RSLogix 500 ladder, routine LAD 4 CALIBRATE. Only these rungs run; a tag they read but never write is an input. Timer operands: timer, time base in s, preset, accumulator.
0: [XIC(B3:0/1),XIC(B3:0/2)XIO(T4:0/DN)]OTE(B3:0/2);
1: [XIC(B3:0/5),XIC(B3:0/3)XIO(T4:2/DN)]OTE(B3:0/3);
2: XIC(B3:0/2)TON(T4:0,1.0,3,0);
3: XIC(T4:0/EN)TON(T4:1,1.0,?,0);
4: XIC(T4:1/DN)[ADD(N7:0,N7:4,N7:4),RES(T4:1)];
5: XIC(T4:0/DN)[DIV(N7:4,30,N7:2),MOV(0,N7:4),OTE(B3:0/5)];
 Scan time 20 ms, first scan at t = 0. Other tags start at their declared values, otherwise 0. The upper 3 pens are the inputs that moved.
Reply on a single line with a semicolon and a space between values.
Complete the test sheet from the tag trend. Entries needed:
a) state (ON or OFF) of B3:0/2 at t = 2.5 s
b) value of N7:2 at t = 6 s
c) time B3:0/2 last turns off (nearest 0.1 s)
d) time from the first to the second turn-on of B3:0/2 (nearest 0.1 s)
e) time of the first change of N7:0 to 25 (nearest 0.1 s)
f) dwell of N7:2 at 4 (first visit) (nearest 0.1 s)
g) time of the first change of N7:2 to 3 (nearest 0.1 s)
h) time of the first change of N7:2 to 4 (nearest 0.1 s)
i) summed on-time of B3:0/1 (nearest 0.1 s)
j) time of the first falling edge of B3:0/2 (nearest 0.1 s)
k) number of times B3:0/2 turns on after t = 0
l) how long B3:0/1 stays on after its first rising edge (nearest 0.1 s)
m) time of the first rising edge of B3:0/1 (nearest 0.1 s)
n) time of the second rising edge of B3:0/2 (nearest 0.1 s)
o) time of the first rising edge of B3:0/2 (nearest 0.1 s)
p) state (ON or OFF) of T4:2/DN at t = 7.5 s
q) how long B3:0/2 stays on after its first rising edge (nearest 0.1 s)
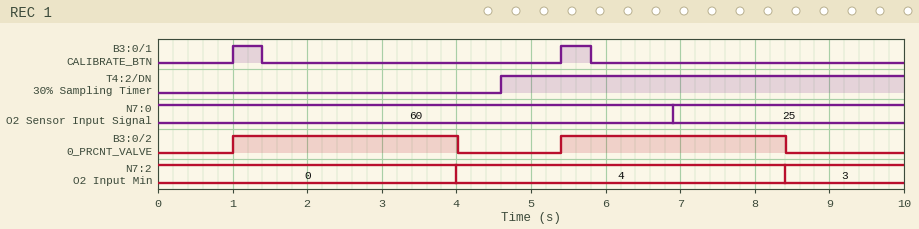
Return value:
ON; 4; 8.4 s; 4.4 s; 6.9 s; 4.4 s; 8.4 s; 4.0 s; 0.8 s; 4.0 s; 2; 0.4 s; 1.0 s; 5.4 s; 1.0 s; ON; 3.0 s
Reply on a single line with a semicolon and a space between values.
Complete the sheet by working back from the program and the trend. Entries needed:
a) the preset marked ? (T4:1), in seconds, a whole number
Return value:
1 s
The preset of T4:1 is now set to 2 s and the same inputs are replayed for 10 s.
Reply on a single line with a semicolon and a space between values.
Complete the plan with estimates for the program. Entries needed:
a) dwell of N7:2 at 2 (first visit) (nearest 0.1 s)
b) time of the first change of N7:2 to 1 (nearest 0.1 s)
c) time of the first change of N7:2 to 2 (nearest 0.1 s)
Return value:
4.4 s; 8.4 s; 4.0 s
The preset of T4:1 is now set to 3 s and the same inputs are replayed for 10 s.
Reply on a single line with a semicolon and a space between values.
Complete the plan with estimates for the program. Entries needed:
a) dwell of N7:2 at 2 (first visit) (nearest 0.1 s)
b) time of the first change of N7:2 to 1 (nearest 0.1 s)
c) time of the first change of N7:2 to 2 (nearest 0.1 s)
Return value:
4.4 s; 8.4 s; 4.0 s
